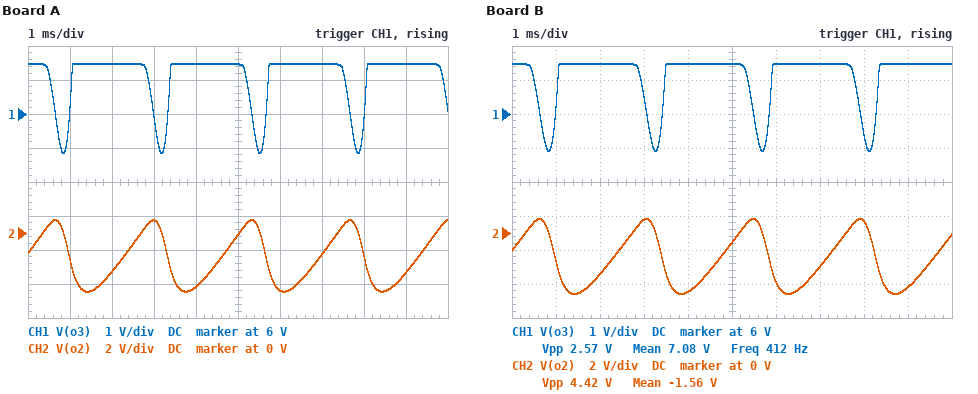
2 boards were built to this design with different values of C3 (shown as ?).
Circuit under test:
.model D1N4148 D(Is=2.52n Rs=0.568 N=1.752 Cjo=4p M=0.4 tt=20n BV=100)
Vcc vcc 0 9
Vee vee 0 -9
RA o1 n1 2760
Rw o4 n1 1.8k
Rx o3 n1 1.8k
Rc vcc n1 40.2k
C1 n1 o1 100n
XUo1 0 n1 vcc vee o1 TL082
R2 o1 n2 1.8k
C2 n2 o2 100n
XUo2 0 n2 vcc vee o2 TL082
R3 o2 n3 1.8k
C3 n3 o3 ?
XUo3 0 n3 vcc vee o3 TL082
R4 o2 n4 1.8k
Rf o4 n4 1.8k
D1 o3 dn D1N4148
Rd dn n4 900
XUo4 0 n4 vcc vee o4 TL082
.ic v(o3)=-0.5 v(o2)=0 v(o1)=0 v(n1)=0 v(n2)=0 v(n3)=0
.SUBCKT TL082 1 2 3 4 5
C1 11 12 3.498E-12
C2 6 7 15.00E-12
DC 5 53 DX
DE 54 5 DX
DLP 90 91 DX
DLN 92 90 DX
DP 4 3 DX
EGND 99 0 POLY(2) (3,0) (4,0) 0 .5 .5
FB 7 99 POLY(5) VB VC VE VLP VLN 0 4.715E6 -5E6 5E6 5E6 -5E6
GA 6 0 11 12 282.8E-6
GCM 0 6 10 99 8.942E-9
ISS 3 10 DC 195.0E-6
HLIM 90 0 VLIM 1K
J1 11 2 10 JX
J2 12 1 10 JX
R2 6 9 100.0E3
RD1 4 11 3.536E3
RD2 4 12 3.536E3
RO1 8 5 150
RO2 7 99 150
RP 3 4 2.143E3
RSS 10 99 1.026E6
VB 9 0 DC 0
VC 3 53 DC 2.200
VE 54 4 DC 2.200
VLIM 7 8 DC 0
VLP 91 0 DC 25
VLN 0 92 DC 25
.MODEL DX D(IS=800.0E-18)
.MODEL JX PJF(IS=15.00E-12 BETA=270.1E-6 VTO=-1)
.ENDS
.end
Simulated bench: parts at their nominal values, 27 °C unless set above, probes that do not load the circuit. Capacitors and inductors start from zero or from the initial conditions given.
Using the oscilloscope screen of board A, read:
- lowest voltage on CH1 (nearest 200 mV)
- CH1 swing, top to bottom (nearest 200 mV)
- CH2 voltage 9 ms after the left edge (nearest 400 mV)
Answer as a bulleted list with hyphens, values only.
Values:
- 4.8 V
- 2.6 V
- -2.4 V
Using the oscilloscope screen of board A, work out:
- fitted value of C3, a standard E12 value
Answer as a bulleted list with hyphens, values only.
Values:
- 47 nF
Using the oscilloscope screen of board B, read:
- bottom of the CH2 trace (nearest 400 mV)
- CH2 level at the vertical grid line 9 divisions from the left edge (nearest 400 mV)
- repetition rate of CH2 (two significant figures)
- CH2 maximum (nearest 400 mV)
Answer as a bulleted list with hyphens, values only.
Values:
- -3.6 V
- -3.2 V
- 410 Hz
- 800 mV
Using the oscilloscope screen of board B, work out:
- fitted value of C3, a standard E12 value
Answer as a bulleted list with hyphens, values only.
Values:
- 56 nF
